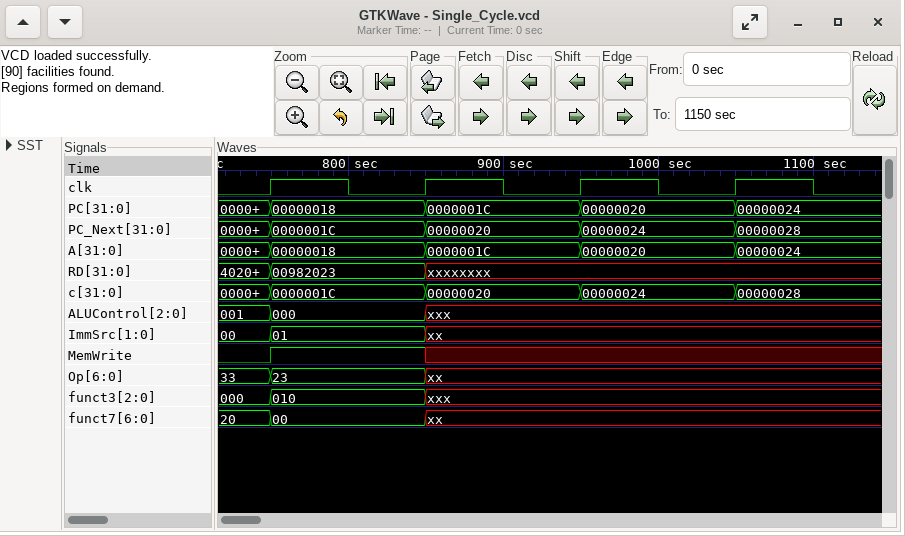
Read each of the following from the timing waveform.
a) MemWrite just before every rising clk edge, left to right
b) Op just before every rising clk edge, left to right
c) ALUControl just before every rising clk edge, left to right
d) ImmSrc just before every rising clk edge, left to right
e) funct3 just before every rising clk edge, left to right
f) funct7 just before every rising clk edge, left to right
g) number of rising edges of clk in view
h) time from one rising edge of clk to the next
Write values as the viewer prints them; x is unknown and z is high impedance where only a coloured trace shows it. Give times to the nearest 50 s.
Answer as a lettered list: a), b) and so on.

a) 0 1 x x
b) 33, 23, xx, xx
c) 001, 000, xxx, xxx
d) 00, 01, xx, xx
e) 000, 010, xxx, xxx
f) 20, 00, xx, xx
g) 4
h) 100 s
